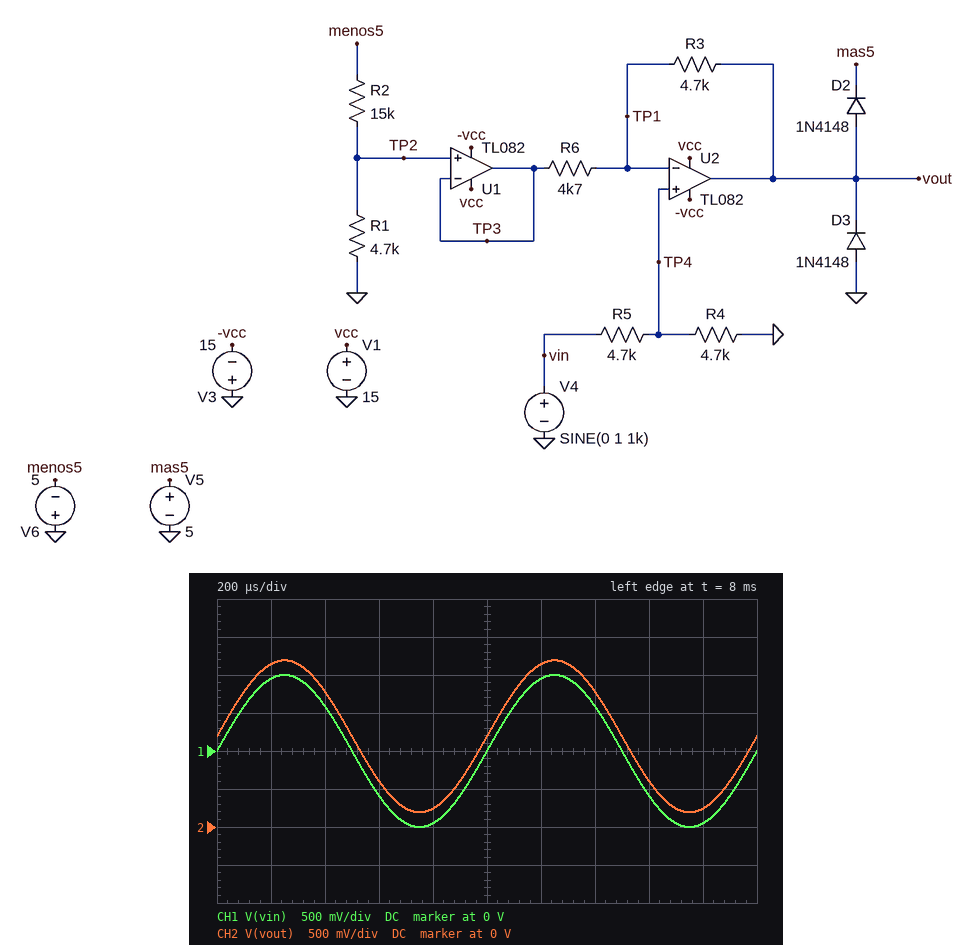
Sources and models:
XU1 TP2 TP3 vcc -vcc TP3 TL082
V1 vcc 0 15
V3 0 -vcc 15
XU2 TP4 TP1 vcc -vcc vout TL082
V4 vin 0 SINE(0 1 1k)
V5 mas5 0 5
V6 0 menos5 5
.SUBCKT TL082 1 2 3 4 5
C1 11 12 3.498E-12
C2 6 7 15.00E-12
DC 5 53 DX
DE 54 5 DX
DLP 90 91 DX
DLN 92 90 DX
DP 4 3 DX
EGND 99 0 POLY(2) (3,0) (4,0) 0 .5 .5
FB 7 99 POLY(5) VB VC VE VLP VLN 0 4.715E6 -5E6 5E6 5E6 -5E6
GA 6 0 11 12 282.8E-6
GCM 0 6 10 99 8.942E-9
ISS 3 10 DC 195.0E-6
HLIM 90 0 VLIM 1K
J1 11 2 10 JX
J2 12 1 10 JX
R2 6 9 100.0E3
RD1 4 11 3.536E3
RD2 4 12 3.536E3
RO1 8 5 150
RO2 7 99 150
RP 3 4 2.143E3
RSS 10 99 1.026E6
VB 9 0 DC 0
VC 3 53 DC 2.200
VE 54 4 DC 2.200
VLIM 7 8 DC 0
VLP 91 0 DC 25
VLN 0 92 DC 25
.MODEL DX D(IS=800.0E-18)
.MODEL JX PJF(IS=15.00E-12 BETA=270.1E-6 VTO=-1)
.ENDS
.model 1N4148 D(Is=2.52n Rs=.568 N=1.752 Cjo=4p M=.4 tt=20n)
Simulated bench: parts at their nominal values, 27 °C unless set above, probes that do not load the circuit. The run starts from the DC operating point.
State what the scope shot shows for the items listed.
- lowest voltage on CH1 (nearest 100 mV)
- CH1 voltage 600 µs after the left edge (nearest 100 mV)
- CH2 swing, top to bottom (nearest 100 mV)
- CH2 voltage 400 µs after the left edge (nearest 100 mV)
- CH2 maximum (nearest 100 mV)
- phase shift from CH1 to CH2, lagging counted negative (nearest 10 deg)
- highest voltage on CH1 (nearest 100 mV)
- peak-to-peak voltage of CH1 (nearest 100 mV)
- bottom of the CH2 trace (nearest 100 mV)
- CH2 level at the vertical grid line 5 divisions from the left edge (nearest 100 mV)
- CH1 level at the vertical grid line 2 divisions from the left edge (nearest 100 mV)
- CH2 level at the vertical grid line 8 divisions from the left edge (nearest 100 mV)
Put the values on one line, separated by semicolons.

-1.0 V; -600 mV; 2.0 V; 1.8 V; 2.2 V; 0 deg; 1.0 V; 2.0 V; 200 mV; 1.2 V; 600 mV; 600 mV
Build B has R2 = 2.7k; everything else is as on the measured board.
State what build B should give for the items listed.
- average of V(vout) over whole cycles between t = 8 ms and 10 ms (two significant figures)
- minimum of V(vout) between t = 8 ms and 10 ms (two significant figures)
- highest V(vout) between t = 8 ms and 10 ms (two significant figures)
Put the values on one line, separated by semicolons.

3.2 V; 2.2 V; 4.2 V
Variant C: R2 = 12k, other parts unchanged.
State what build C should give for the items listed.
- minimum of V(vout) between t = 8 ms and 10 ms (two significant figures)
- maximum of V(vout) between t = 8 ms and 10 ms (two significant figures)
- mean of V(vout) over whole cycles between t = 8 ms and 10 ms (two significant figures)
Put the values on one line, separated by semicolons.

410 mV; 2.4 V; 1.4 V
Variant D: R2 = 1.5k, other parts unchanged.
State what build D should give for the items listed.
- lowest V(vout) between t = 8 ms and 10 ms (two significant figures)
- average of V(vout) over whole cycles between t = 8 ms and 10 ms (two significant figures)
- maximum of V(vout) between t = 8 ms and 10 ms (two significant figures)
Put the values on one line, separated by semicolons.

2.8 V; 3.8 V; 4.8 V
